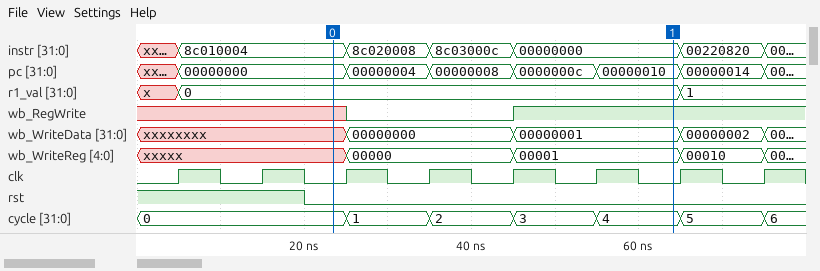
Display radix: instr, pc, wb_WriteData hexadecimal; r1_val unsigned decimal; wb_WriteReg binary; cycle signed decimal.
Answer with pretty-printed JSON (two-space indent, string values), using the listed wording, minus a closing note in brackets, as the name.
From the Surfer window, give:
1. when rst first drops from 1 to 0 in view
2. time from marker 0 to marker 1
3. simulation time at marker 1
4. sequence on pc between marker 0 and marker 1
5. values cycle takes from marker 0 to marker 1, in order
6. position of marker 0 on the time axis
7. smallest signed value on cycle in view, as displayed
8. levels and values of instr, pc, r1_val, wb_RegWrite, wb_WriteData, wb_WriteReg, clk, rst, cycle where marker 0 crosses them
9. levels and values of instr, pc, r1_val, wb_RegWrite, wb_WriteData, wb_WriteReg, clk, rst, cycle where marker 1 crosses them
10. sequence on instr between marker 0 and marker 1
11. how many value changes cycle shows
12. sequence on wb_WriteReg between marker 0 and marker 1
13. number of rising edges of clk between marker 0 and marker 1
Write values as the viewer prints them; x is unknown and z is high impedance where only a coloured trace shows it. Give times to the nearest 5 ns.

{
  "when rst first drops from 1 to 0 in view": "20 ns",
  "time from marker 0 to marker 1": "40 ns",
  "simulation time at marker 1": "65 ns",
  "sequence on pc between marker 0 and marker 1": "00000000, 00000004, 00000008, 0000000c, 00000010",
  "values cycle takes from marker 0 to marker 1, in order": "0, 1, 2, 3, 4",
  "position of marker 0 on the time axis": "25 ns",
  "smallest signed value on cycle in view, as displayed": "0",
  "levels and values of instr, pc, r1_val, wb_RegWrite, wb_WriteData, wb_WriteReg, clk, rst, cycle where marker 0 crosses them": "instr=8c010004, pc=00000000, r1_val=0, wb_RegWrite=x, wb_WriteData=xxxxxxxx, wb_WriteReg=xxxxx, clk=0, rst=0, cycle=0",
  "levels and values of instr, pc, r1_val, wb_RegWrite, wb_WriteData, wb_WriteReg, clk, rst, cycle where marker 1 crosses them": "instr=00000000, pc=00000010, r1_val=0, wb_RegWrite=1, wb_WriteData=00000001, wb_WriteReg=00001, clk=0, rst=0, cycle=4",
  "sequence on instr between marker 0 and marker 1": "8c010004, 8c020008, 8c03000c, 00000000",
  "how many value changes cycle shows": "6",
  "sequence on wb_WriteReg between marker 0 and marker 1": "xxxxx, 00000, 00001",
  "number of rising edges of clk between marker 0 and marker 1": "4"
}
